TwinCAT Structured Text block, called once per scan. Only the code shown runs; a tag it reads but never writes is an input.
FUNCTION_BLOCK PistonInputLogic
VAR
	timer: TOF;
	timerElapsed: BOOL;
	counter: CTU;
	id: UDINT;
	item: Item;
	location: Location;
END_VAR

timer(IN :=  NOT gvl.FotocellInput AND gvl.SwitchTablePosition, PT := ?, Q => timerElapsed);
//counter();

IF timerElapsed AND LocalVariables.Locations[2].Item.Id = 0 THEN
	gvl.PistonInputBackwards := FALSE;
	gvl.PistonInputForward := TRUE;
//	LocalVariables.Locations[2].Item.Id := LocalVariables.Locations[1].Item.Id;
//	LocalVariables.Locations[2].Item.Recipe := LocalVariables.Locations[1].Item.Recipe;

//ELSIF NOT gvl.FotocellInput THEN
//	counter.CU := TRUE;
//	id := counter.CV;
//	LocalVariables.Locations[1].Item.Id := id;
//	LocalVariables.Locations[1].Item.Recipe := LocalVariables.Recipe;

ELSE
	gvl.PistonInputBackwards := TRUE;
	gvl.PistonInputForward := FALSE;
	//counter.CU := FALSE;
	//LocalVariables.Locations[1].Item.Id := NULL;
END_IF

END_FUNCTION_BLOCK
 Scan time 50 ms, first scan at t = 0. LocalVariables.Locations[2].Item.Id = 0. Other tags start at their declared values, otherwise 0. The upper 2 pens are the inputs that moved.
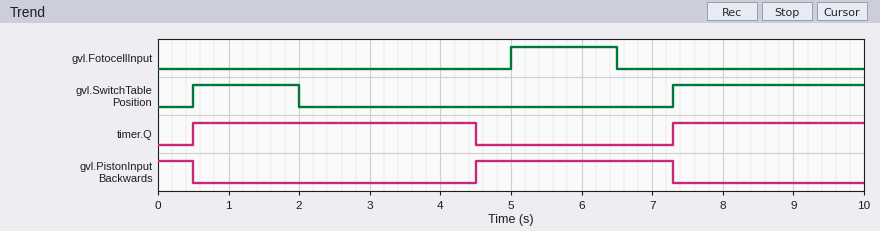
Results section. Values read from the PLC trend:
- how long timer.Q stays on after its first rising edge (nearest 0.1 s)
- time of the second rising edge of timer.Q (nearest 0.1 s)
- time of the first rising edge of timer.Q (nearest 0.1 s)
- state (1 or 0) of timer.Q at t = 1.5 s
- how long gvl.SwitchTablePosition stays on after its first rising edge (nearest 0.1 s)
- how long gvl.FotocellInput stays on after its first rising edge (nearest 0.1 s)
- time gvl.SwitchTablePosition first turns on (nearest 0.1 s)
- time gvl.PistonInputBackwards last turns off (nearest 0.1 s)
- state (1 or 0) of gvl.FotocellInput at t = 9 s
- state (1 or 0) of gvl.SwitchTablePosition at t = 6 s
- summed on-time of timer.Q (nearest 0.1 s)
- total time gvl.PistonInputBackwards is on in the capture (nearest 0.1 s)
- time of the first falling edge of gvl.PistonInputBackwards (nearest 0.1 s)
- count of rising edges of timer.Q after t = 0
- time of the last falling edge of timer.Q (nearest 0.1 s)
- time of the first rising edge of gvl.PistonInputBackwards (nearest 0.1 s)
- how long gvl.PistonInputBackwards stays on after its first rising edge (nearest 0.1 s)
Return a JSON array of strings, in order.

["4.0 s", "7.3 s", "0.5 s", "1", "1.5 s", "1.5 s", "0.5 s", "7.3 s", "0", "0", "6.7 s", "3.3 s", "0.5 s", "2", "4.5 s", "4.5 s", "2.8 s"]
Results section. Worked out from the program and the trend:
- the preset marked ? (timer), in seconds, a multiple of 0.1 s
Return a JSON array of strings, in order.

["2.5 s"]
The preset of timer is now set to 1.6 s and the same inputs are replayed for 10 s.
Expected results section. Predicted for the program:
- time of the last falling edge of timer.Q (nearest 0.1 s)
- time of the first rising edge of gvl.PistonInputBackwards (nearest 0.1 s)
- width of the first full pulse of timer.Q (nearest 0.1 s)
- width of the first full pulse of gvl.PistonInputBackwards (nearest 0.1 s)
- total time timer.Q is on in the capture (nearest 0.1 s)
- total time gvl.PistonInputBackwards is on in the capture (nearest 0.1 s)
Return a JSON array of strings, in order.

["3.6 s", "3.6 s", "3.1 s", "3.7 s", "5.8 s", "4.2 s"]
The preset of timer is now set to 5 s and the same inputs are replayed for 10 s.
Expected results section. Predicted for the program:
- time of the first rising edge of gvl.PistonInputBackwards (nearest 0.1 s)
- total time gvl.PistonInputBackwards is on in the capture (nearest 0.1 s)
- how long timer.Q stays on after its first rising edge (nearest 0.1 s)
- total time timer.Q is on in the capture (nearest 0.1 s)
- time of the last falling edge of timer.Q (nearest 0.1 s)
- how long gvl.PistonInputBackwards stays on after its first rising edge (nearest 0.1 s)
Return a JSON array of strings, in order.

["7.0 s", "0.8 s", "6.5 s", "9.2 s", "7.0 s", "0.3 s"]
